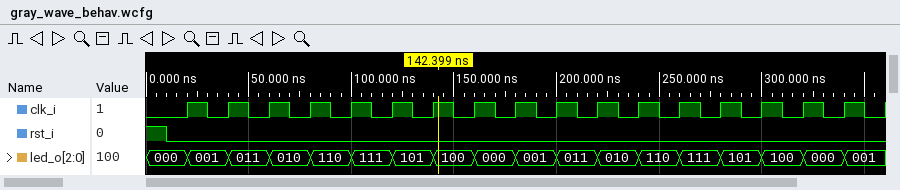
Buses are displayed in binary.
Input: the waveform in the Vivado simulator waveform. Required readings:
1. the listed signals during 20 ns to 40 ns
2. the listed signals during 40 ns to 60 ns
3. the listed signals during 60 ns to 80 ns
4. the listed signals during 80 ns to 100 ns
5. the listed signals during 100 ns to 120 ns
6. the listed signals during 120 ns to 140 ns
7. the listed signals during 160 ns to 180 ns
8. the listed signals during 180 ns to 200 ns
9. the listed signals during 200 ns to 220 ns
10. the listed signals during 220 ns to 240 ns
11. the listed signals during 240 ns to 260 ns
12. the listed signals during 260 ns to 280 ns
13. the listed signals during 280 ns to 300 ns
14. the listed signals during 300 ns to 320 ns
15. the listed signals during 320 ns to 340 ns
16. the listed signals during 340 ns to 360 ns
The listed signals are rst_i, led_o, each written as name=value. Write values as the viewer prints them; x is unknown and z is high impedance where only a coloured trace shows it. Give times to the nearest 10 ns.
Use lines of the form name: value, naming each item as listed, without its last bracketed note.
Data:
the listed signals during 20 ns to 40 ns: rst_i=0, led_o=001
the listed signals during 40 ns to 60 ns: rst_i=0, led_o=011
the listed signals during 60 ns to 80 ns: rst_i=0, led_o=010
the listed signals during 80 ns to 100 ns: rst_i=0, led_o=110
the listed signals during 100 ns to 120 ns: rst_i=0, led_o=111
the listed signals during 120 ns to 140 ns: rst_i=0, led_o=101
the listed signals during 160 ns to 180 ns: rst_i=0, led_o=000
the listed signals during 180 ns to 200 ns: rst_i=0, led_o=001
the listed signals during 200 ns to 220 ns: rst_i=0, led_o=011
the listed signals during 220 ns to 240 ns: rst_i=0, led_o=010
the listed signals during 240 ns to 260 ns: rst_i=0, led_o=110
the listed signals during 260 ns to 280 ns: rst_i=0, led_o=111
the listed signals during 280 ns to 300 ns: rst_i=0, led_o=101
the listed signals during 300 ns to 320 ns: rst_i=0, led_o=100
the listed signals during 320 ns to 340 ns: rst_i=0, led_o=000
the listed signals during 340 ns to 360 ns: rst_i=0, led_o=001
